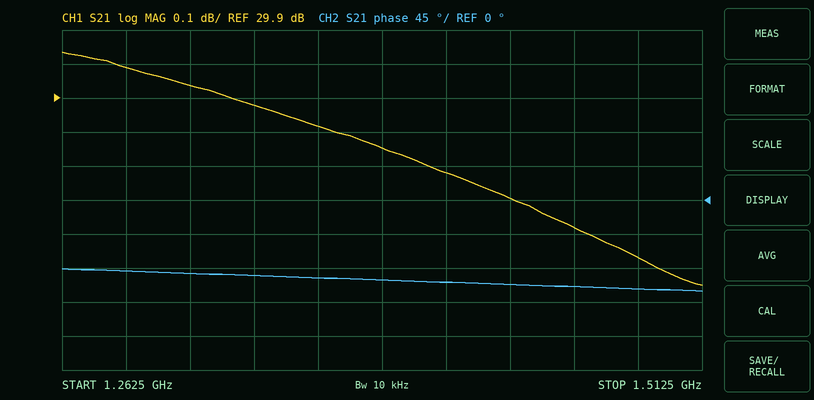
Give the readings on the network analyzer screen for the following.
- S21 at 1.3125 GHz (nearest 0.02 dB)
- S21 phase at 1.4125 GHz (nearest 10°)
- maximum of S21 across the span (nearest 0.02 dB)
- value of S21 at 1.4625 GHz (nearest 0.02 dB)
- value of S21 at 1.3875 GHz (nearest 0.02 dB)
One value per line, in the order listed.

29.94 dB
-110°
30.04 dB
29.52 dB
29.76 dB
